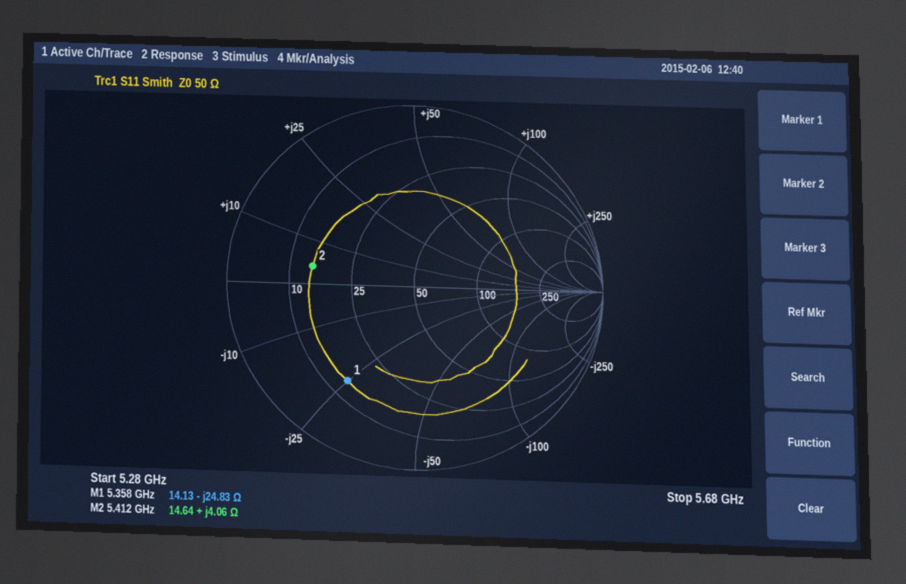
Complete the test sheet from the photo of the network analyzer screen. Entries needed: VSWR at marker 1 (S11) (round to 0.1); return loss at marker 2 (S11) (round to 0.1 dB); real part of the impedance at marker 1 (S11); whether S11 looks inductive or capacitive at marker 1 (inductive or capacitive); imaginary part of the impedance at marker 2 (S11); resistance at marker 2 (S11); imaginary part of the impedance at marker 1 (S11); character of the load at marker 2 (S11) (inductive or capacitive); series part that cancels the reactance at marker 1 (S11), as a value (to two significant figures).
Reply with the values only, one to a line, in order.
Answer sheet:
4.5
5.2 dB
14.13 Ω
capacitive
+4.06 Ω
14.64 Ω
-24.83 Ω
inductive
740 pH
